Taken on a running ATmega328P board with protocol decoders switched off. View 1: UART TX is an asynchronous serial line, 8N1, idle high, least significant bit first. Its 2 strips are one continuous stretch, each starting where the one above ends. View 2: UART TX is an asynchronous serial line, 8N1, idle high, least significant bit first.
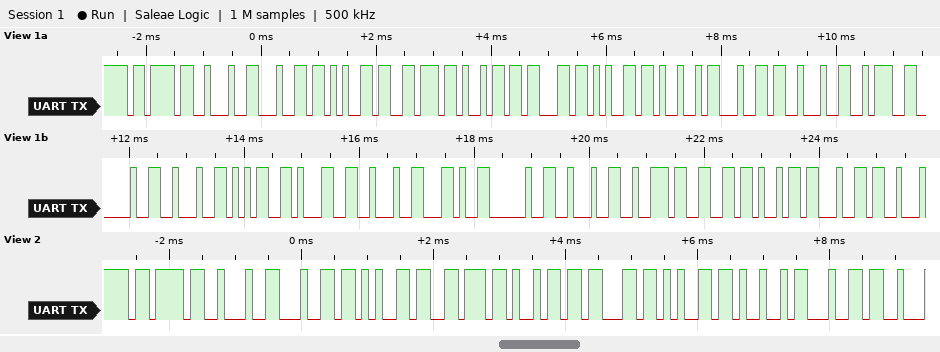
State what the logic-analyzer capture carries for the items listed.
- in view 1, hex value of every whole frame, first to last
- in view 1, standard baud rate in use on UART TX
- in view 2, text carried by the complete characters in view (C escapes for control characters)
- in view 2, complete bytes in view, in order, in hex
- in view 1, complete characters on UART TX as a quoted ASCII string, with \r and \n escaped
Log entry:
0x7B 0x22 0x64 0x65 0x76 0x69 0x63 0x65 0x49 0x64 0x22 0x3A 0x20 0x22 0x35 0x31 0x22 0x2C 0x20 0x22 0x72 0x66 0x69 0x64
9600 baud
"{\"deviceId"
0x7B 0x22 0x64 0x65 0x76 0x69 0x63 0x65 0x49 0x64
"{\"deviceId\": \"51\", \"rfid"
